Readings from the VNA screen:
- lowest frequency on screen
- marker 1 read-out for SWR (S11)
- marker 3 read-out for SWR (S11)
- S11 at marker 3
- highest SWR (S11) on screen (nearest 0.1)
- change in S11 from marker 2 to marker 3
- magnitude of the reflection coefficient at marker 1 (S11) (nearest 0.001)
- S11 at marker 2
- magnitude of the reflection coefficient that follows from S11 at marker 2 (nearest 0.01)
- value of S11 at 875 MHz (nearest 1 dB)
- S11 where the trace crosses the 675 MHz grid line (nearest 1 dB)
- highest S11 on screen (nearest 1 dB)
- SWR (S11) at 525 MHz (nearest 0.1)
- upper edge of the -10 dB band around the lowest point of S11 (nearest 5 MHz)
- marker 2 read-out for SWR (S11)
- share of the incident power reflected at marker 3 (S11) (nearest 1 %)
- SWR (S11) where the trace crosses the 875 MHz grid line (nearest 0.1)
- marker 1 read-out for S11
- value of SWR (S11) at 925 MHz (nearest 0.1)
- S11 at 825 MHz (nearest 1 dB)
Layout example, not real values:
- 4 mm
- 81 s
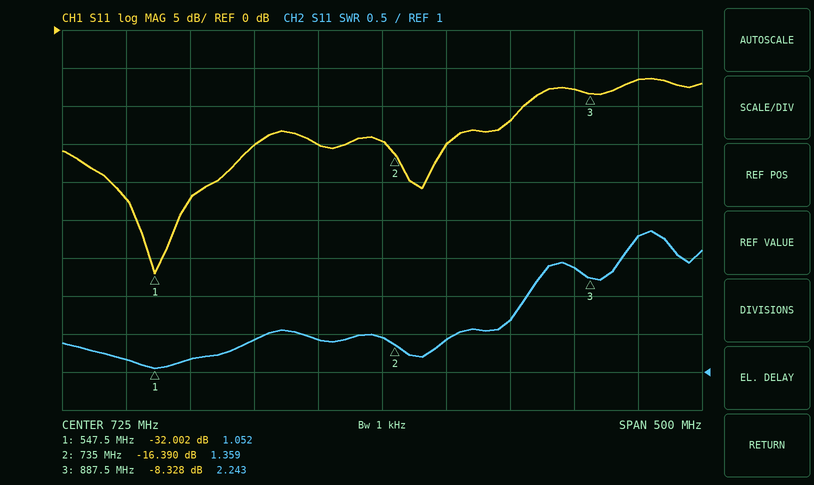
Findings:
- 475 MHz
- 1.052
- 2.243
- -8.328 dB
- 2.9
- 8.062 dB
- 0.025
- -16.390 dB
- 0.15
- -8 dB
- -15 dB
- -6 dB
- 1.2
- 835 MHz
- 1.359
- 15 %
- 2.4
- -32.002 dB
- 2.8
- -12 dB
